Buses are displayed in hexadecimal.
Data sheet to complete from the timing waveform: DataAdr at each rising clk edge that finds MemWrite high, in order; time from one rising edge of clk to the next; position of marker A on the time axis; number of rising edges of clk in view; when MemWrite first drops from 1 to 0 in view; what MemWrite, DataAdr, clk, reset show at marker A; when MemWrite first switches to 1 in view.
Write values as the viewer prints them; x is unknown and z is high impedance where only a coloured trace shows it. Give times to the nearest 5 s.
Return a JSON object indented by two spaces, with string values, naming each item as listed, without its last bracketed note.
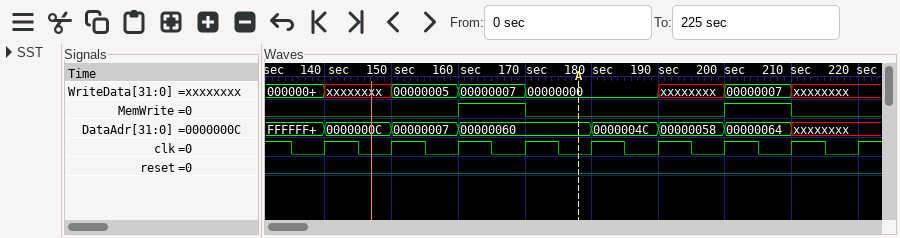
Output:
{
  "DataAdr at each rising clk edge that finds MemWrite high, in order": "00000060, 00000064",
  "time from one rising edge of clk to the next": "10 s",
  "position of marker A on the time axis": "180 s",
  "number of rising edges of clk in view": "9",
  "when MemWrite first drops from 1 to 0 in view": "170 s",
  "what MemWrite, DataAdr, clk, reset show at marker A": "MemWrite=0, DataAdr=00000060, clk=0, reset=0",
  "when MemWrite first switches to 1 in view": "160 s"
}
